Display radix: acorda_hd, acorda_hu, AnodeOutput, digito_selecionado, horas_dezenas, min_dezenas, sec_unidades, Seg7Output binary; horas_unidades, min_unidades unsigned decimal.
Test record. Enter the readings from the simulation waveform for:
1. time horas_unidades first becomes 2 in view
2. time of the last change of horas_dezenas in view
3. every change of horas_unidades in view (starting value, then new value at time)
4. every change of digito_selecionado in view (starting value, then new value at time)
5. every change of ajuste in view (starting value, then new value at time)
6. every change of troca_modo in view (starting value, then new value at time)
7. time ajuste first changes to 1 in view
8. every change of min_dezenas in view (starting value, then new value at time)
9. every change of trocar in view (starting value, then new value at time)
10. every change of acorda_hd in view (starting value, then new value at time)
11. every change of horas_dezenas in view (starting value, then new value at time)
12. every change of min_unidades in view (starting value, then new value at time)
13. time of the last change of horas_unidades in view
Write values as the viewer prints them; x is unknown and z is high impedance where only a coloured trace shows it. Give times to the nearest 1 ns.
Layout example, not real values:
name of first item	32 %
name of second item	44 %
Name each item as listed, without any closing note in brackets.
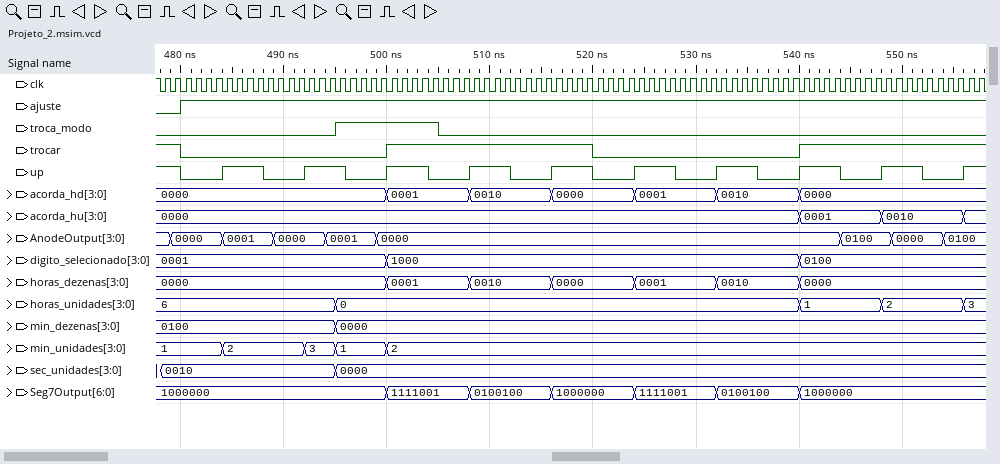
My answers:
time horas_unidades first becomes 2 in view	548 ns
time of the last change of horas_dezenas in view	540 ns
every change of horas_unidades in view	6, 0 at 495 ns, 1 at 540 ns, 2 at 548 ns, 3 at 556 ns
every change of digito_selecionado in view	0001, 1000 at 500 ns, 0100 at 540 ns
every change of ajuste in view	0, 1 at 480 ns
every change of troca_modo in view	0, 1 at 495 ns, 0 at 505 ns
time ajuste first changes to 1 in view	480 ns
every change of min_dezenas in view	0100, 0000 at 495 ns
every change of trocar in view	1, 0 at 480 ns, 1 at 500 ns, 0 at 520 ns, 1 at 540 ns
every change of acorda_hd in view	0000, 0001 at 500 ns, 0010 at 508 ns, 0000 at 516 ns, 0001 at 524 ns, 0010 at 532 ns, 0000 at 540 ns
every change of horas_dezenas in view	0000, 0001 at 500 ns, 0010 at 508 ns, 0000 at 516 ns, 0001 at 524 ns, 0010 at 532 ns, 0000 at 540 ns
every change of min_unidades in view	1, 2 at 484 ns, 3 at 492 ns, 1 at 495 ns, 2 at 500 ns
time of the last change of horas_unidades in view	556 ns
